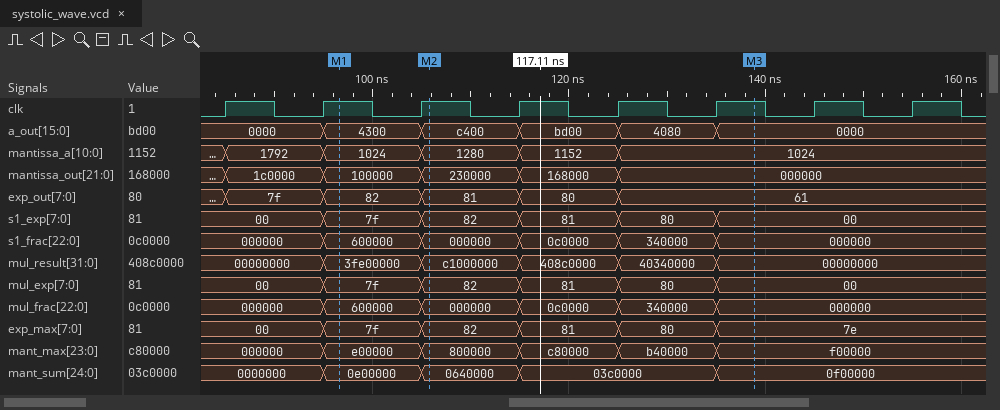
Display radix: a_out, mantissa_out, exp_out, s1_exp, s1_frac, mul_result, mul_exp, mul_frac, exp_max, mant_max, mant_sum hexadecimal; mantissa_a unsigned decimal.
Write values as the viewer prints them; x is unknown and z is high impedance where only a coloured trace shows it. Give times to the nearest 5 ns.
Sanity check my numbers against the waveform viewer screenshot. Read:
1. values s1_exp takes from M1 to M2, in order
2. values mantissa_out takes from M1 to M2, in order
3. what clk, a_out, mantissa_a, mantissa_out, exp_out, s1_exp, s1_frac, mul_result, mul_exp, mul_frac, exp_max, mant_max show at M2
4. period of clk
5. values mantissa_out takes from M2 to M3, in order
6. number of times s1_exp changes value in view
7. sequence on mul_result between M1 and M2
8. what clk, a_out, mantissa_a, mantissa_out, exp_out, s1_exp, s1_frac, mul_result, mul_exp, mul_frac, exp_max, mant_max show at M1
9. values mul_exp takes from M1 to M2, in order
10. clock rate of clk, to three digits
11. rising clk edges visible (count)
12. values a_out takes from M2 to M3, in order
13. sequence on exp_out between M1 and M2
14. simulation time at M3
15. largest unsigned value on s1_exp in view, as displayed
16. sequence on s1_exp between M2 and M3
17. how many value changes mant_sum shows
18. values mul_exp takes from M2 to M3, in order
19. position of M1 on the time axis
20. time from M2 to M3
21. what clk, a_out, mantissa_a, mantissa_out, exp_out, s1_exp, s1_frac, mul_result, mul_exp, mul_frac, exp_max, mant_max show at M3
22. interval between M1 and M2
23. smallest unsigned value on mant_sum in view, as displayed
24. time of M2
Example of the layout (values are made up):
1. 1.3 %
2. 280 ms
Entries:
1. 7f, 82
2. 100000, 230000
3. clk=1, a_out=c400, mantissa_a=1280, mantissa_out=230000, exp_out=81, s1_exp=82, s1_frac=000000, mul_result=c1000000, mul_exp=82, mul_frac=000000, exp_max=82, mant_max=800000
4. 10 ns
5. 230000, 168000, 000000
6. 5
7. 3fe00000, c1000000
8. clk=1, a_out=4300, mantissa_a=1024, mantissa_out=100000, exp_out=82, s1_exp=7f, s1_frac=600000, mul_result=3fe00000, mul_exp=7f, mul_frac=600000, exp_max=7f, mant_max=e00000
9. 7f, 82
10. 100 MHz
11. 8
12. c400, bd00, 4080, 0000
13. 82, 81
14. 140 ns
15. 82
16. 82, 81, 80, 00
17. 4
18. 82, 81, 80, 00
19. 95 ns
20. 35 ns
21. clk=1, a_out=0000, mantissa_a=1024, mantissa_out=000000, exp_out=61, s1_exp=00, s1_frac=000000, mul_result=00000000, mul_exp=00, mul_frac=000000, exp_max=7e, mant_max=f00000
22. 10 ns
23. 0000000
24. 105 ns
